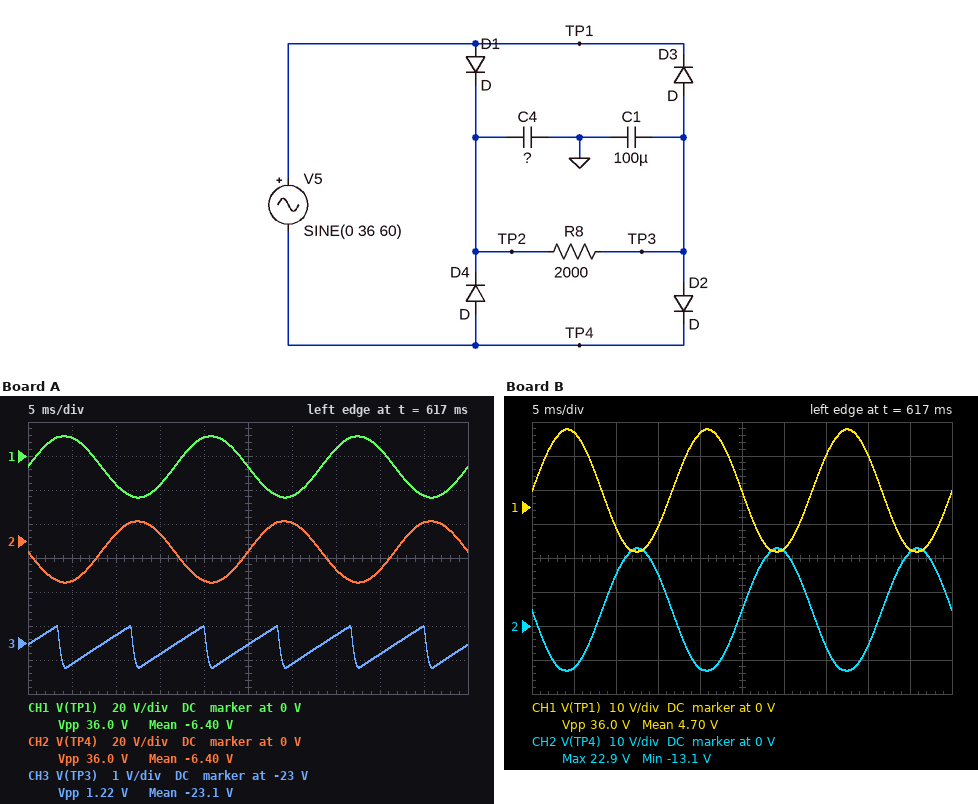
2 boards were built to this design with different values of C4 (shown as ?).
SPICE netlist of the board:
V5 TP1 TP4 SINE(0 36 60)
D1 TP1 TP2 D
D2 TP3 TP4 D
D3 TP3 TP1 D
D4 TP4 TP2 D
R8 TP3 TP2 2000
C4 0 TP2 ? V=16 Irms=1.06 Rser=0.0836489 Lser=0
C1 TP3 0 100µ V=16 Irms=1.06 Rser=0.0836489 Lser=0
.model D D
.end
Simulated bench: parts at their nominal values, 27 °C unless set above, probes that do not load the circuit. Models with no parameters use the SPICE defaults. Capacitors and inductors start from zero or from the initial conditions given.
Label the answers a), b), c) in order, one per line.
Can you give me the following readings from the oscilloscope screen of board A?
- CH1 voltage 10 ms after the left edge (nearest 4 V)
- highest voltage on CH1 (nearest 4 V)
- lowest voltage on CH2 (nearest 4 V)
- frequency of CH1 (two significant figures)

a) -16 V
b) 12 V
c) -24 V
d) 60 Hz
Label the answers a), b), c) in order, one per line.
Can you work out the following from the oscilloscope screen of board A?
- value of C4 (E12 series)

a) 220 µF
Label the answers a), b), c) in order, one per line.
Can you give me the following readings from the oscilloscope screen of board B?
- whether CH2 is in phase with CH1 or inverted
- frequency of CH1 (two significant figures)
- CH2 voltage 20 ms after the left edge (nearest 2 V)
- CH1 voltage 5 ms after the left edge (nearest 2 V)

a) inverted
b) 60 Hz
c) -12 V
d) 22 V
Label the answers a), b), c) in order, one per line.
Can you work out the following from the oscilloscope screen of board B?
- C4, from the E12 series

a) 56 µF
